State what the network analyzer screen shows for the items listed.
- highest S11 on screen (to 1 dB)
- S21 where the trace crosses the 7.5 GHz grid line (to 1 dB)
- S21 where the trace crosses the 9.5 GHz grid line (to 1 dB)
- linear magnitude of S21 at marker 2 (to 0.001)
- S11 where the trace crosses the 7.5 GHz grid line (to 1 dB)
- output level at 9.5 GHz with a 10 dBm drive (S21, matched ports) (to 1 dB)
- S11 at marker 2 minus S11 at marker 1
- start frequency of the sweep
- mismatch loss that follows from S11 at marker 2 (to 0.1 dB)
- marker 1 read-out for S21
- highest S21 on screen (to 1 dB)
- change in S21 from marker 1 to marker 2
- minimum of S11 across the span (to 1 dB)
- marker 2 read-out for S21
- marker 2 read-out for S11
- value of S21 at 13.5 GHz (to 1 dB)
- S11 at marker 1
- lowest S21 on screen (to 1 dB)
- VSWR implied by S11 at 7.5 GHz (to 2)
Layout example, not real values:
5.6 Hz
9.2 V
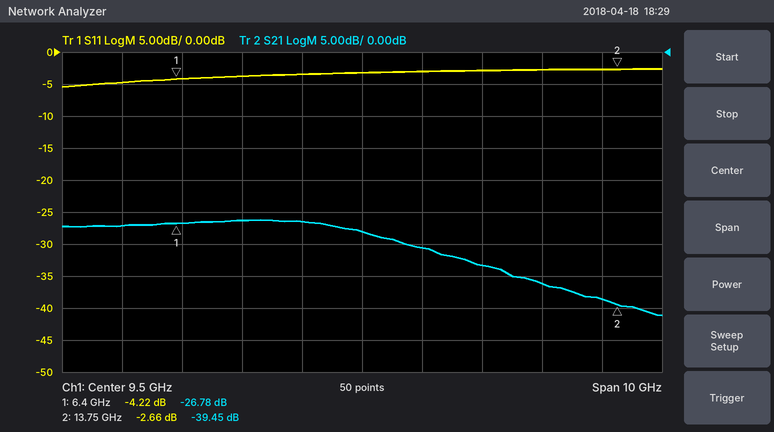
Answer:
-3 dB
-26 dB
-28 dB
0.011
-4 dB
-18 dBm
1.56 dB
4.5 GHz
3.4 dB
-26.78 dB
-26 dB
-12.67 dB
-5 dB
-39.45 dB
-2.66 dB
-39 dB
-4.22 dB
-41 dB
4
